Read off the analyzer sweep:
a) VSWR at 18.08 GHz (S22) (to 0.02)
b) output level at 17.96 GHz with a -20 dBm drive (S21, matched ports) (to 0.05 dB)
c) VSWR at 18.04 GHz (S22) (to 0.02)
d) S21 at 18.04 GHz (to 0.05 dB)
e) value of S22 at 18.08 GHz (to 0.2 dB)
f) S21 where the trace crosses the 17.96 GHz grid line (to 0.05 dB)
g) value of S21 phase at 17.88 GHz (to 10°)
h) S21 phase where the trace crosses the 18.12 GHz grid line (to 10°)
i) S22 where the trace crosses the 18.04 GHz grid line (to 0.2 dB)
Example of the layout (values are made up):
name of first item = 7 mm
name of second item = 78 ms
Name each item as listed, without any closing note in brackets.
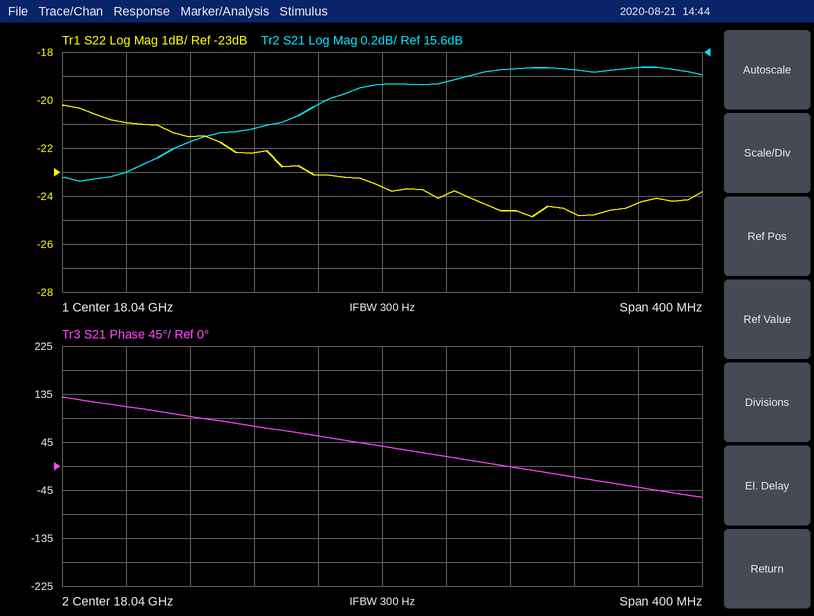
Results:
VSWR at 18.08 GHz (S22) = 1.14
output level at 17.96 GHz with a -20 dBm drive (S21, matched ports) = -5.05 dBm
VSWR at 18.04 GHz (S22) = 1.14
S21 at 18.04 GHz = 15.35 dB
value of S22 at 18.08 GHz = -24.0 dB
S21 where the trace crosses the 17.96 GHz grid line = 14.95 dB
value of S21 phase at 17.88 GHz = 110°
S21 phase where the trace crosses the 18.12 GHz grid line = 0°
S22 where the trace crosses the 18.04 GHz grid line = -23.6 dB
